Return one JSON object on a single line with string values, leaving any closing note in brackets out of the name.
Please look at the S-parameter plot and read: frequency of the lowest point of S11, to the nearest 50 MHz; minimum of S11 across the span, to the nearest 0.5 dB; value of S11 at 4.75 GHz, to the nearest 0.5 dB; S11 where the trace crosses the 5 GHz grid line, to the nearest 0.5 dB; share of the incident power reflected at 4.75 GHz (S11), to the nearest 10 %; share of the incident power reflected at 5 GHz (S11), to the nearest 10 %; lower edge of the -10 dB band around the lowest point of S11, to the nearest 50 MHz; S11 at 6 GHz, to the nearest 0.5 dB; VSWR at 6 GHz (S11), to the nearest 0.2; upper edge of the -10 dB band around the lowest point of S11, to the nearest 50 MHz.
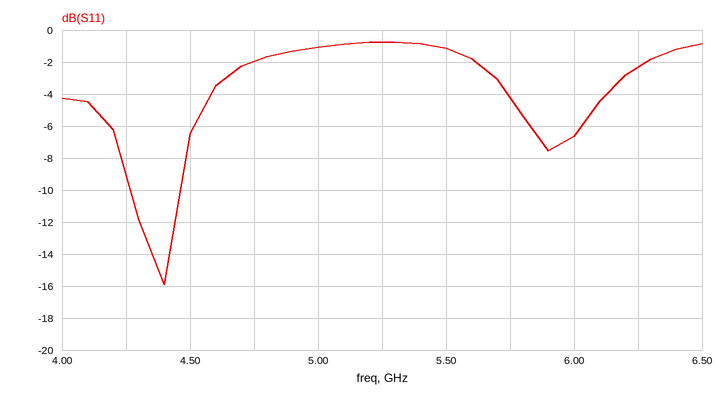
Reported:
{"frequency of the lowest point of S11, to the nearest 50 MHz": "4.40 GHz", "minimum of S11 across the span, to the nearest 0.5 dB": "-16.0 dB", "value of S11 at 4.75 GHz, to the nearest 0.5 dB": "-2.0 dB", "S11 where the trace crosses the 5 GHz grid line, to the nearest 0.5 dB": "-1.0 dB", "share of the incident power reflected at 4.75 GHz (S11), to the nearest 10 %": "60 %", "share of the incident power reflected at 5 GHz (S11), to the nearest 10 %": "80 %", "lower edge of the -10 dB band around the lowest point of S11, to the nearest 50 MHz": "4.25 GHz", "S11 at 6 GHz, to the nearest 0.5 dB": "-6.5 dB", "VSWR at 6 GHz (S11), to the nearest 0.2": "2.8", "upper edge of the -10 dB band around the lowest point of S11, to the nearest 50 MHz": "4.45 GHz"}
